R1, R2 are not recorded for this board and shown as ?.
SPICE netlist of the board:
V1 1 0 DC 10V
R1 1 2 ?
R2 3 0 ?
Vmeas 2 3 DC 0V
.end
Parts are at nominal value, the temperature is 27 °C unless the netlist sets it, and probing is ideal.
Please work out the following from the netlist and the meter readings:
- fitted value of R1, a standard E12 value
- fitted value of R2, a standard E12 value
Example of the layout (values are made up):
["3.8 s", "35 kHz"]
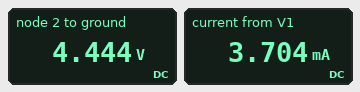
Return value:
["1.5 kΩ", "1.2 kΩ"]
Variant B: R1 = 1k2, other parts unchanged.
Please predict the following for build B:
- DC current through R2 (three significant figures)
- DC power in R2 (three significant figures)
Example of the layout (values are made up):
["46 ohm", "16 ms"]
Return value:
["4.17 mA", "20.8 mW"]
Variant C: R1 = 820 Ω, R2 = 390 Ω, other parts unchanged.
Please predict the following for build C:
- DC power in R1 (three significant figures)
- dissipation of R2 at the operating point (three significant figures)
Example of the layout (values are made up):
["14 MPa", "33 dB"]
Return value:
["56.0 mW", "26.6 mW"]
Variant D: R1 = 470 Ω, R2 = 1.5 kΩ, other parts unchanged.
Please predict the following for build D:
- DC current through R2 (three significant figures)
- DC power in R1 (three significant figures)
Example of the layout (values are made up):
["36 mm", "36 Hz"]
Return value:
["5.08 mA", "12.1 mW"]
